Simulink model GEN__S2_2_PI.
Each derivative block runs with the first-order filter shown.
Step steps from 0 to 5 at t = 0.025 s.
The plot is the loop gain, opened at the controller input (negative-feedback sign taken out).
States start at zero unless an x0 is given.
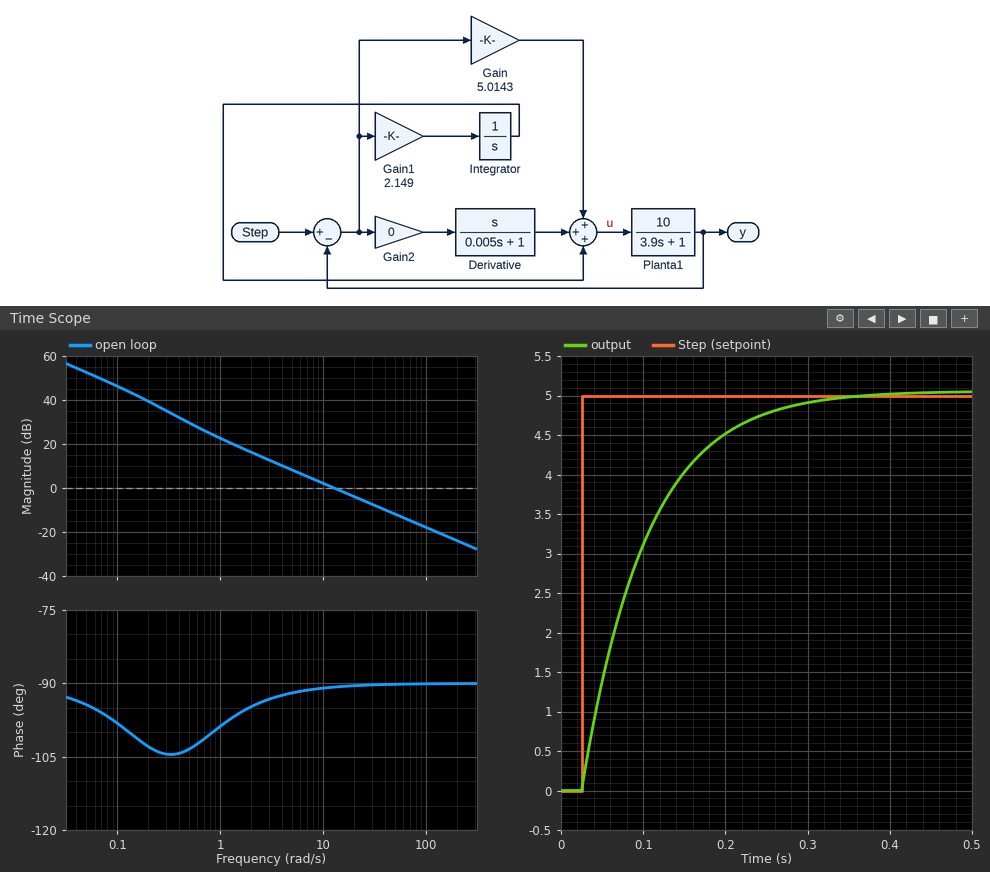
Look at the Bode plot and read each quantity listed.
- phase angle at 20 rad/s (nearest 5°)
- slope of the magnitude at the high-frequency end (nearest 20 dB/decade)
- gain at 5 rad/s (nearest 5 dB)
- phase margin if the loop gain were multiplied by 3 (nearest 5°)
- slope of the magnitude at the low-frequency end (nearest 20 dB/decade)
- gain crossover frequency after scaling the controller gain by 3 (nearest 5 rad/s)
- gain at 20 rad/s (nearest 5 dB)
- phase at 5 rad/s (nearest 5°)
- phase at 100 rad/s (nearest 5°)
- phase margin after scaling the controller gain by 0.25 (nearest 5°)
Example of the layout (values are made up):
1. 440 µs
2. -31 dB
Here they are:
1. -90°
2. -20 dB/decade
3. 10 dB
4. 90°
5. -20 dB/decade
6. 40 rad/s
7. -5 dB
8. -90°
9. -90°
10. 85°
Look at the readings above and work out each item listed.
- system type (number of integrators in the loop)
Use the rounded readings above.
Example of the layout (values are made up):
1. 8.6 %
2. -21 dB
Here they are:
1. 1
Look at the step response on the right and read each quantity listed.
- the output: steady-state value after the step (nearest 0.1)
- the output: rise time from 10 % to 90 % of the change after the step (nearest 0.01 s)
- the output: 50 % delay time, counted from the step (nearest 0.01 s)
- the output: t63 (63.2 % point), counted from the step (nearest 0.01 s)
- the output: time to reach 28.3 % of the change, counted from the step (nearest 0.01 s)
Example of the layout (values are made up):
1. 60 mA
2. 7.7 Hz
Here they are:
1. 5.0
2. 0.17 s
3. 0.05 s
4. 0.08 s
5. 0.03 s
